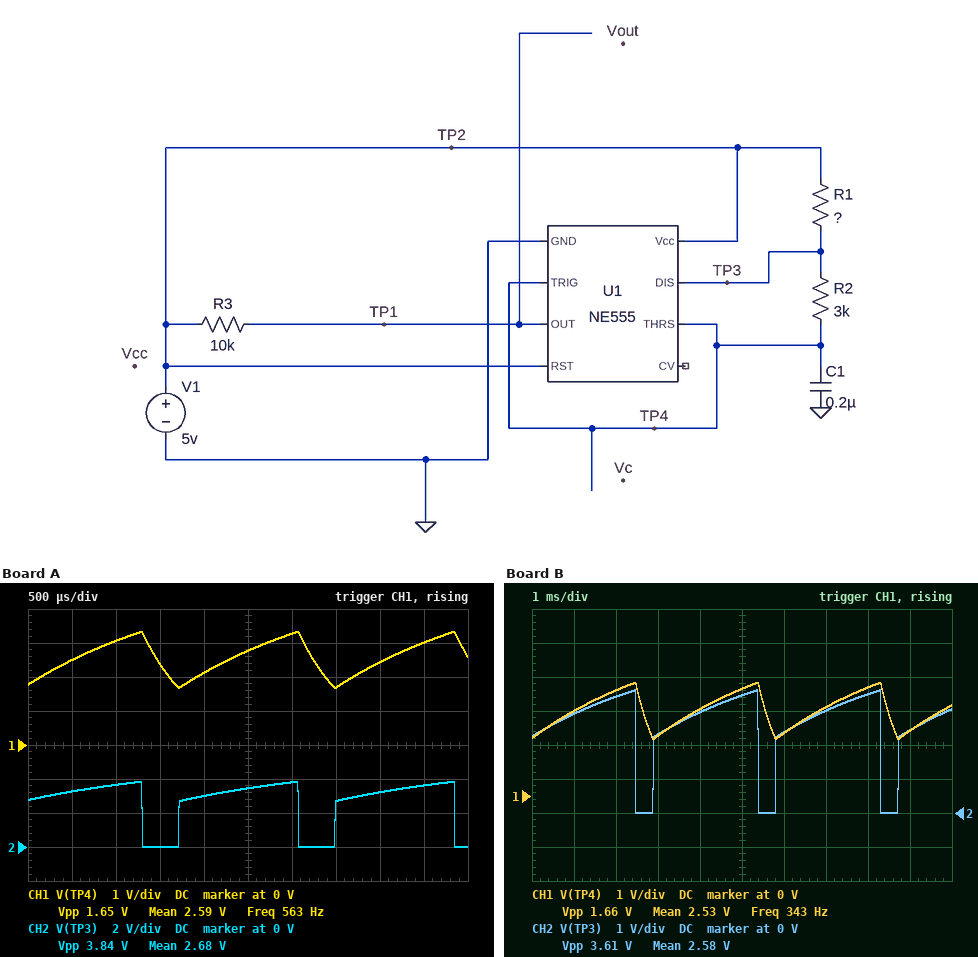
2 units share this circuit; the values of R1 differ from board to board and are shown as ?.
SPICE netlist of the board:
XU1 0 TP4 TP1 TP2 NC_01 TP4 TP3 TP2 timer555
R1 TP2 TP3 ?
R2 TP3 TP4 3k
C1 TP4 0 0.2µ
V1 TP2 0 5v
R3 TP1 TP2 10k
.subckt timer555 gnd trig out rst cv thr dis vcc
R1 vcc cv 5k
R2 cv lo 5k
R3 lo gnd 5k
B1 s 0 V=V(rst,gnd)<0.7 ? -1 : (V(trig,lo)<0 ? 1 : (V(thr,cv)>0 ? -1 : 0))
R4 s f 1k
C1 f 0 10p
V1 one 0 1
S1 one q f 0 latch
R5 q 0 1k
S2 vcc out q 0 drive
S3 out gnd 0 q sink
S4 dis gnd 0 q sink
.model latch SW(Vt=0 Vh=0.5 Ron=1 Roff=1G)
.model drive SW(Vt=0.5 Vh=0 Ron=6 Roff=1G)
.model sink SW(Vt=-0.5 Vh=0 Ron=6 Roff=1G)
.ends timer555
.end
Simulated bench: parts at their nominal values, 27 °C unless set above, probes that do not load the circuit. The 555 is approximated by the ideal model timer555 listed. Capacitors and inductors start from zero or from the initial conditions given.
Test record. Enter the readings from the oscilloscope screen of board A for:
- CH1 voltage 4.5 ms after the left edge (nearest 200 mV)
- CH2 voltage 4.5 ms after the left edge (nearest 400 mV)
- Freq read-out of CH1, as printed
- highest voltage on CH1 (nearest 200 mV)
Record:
3.0 V
3.6 V
563 Hz
3.4 V
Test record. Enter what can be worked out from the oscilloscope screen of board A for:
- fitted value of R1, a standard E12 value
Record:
6.8 kΩ
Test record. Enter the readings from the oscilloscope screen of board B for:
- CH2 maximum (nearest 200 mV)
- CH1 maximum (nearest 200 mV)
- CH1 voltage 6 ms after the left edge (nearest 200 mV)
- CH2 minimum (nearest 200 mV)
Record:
3.6 V
3.4 V
1.8 V
0 V
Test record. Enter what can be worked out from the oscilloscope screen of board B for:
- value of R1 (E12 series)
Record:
15 kΩ
